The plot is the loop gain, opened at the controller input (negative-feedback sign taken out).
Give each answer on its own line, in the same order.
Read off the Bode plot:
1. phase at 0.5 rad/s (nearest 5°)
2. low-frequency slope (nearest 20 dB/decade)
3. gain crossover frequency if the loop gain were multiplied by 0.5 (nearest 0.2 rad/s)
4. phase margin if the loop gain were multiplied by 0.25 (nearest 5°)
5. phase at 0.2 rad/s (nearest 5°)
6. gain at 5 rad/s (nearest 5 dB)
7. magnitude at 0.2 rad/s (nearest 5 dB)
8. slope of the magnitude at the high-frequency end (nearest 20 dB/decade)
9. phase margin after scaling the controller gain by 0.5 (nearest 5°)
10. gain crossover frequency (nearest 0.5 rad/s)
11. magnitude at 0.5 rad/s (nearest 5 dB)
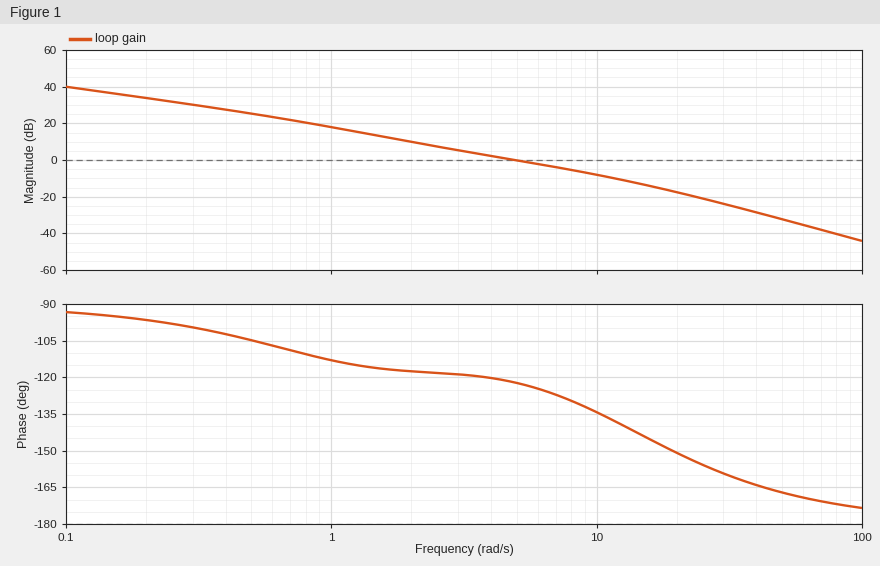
-105°
-20 dB/decade
2.8 rad/s
65°
-95°
0 dB
35 dB
-40 dB/decade
60°
5.0 rad/s
25 dB
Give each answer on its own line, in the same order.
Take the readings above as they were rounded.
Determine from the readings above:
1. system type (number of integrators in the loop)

1
